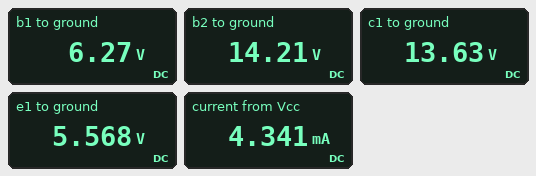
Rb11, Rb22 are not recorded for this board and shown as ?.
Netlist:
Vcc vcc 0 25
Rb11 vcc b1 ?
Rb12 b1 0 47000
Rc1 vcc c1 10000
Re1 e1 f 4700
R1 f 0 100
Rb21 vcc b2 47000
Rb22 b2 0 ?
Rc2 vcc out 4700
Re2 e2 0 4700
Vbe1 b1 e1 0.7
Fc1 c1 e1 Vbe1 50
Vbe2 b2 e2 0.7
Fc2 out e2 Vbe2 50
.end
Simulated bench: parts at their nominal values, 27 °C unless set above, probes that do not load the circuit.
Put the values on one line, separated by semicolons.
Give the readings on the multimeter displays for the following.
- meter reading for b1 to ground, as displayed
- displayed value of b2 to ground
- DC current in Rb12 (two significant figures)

6.27 V; 14.21 V; 130 µA
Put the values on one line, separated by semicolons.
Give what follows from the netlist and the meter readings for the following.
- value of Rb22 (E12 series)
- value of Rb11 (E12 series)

82 kΩ; 120 kΩ
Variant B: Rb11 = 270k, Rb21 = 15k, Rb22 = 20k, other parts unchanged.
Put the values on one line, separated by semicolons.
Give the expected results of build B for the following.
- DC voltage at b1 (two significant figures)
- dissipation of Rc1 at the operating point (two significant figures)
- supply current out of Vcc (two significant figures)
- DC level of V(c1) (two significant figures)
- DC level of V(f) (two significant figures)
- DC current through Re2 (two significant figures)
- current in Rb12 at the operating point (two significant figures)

3.3 V; 2.8 mW; 4.1 mA; 20 V; 54 mV; 2.8 mA; 70 µA
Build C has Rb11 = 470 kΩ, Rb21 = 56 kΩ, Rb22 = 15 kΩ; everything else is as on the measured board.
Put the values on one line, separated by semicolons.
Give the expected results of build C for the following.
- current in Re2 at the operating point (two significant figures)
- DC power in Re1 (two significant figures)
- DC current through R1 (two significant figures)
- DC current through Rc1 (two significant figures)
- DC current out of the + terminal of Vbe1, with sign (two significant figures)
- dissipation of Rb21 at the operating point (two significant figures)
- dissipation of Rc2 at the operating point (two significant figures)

930 µA; 370 µW; 280 µA; 270 µA; -5.5 µA; 7.1 mW; 3.9 mW
